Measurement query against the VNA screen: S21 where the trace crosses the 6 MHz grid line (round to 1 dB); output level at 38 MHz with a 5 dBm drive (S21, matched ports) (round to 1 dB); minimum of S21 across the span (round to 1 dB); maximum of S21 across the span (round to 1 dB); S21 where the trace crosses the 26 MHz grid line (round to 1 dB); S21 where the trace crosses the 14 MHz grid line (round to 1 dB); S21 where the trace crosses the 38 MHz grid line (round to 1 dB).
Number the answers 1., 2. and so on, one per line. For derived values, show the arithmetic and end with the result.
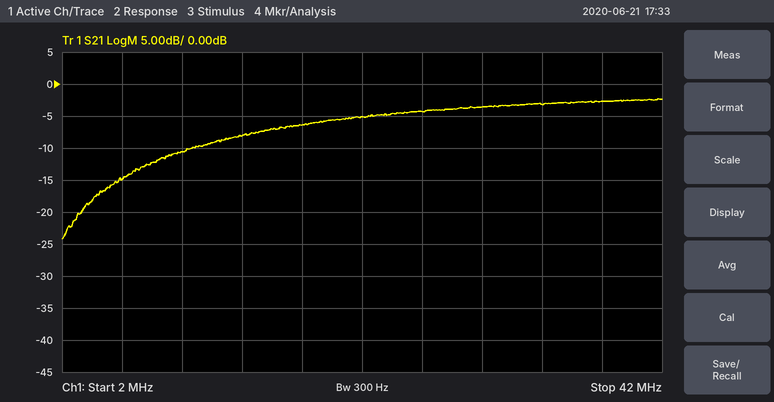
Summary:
1. -15 dB
2. 5 dBm + (-3 dB) = 2 dBm
3. -24 dB
4. -2 dB
5. -4 dB
6. -8 dB
7. -3 dB
